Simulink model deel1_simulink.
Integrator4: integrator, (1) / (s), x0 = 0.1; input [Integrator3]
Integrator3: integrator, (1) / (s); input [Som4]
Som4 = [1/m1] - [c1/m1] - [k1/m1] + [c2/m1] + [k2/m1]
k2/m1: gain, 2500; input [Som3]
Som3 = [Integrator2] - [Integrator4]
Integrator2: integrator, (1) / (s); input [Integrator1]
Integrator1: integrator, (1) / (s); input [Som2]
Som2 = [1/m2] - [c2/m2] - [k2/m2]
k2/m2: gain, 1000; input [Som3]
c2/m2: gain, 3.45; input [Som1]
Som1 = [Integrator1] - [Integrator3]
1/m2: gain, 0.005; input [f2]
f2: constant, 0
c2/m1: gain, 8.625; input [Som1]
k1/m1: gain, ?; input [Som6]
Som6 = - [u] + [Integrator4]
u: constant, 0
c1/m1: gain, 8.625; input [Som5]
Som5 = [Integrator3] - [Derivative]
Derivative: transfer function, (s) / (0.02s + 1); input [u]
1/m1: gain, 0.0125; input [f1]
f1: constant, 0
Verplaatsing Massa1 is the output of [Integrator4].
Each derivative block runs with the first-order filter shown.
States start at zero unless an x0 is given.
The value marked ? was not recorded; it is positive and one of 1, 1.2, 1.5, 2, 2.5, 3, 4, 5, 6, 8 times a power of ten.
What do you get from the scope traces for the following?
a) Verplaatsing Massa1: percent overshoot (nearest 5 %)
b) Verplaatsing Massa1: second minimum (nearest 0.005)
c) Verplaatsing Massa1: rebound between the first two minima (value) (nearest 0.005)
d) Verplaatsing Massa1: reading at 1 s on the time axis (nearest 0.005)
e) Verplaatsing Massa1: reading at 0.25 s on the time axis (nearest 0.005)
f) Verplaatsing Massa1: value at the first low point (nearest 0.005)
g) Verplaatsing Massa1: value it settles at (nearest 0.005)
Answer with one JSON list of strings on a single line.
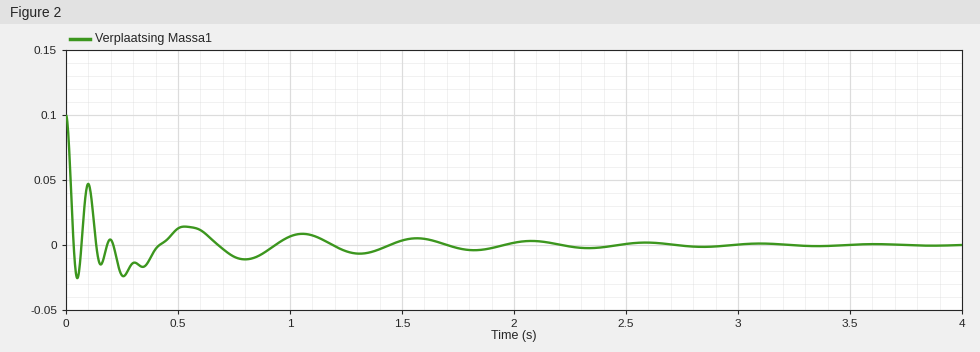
["25 %", "-0.015", "0.045", "0.005", "-0.025", "-0.025", "0.000"]
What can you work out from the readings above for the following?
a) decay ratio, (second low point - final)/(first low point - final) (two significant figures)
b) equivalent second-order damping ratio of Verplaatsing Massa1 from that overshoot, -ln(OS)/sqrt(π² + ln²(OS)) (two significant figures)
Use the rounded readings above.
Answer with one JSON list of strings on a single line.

["0.60", "0.40"]
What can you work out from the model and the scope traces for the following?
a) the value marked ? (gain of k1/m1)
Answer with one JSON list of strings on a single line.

["600"]
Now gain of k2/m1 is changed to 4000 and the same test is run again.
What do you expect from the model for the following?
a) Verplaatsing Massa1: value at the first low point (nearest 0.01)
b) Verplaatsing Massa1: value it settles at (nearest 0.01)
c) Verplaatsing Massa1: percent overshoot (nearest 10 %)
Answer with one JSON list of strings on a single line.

["-0.04", "0.00", "40 %"]
